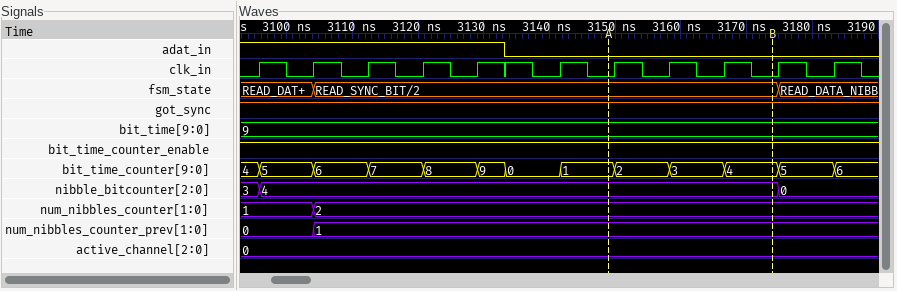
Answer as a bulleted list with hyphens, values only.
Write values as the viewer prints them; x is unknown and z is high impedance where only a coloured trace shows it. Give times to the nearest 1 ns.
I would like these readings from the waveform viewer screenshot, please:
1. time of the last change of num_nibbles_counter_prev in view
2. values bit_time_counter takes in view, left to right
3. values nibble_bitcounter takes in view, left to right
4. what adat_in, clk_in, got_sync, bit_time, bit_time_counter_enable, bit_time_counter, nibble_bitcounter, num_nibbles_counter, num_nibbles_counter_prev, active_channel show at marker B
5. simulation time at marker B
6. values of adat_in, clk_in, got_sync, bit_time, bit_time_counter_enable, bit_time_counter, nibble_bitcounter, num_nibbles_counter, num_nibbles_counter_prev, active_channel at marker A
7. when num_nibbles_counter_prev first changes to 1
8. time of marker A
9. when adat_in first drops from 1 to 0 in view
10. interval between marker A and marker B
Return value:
- 3104 ns
- 4, 5, 6, 7, 8, 9, 0, 1, 2, 3, 4, 5, 6
- 3, 4, 0
- adat_in=0, clk_in=0, got_sync=1, bit_time=9, bit_time_counter_enable=1, bit_time_counter=4, nibble_bitcounter=4, num_nibbles_counter=2, num_nibbles_counter_prev=1, active_channel=0
- 3174 ns
- adat_in=0, clk_in=0, got_sync=1, bit_time=9, bit_time_counter_enable=1, bit_time_counter=1, nibble_bitcounter=4, num_nibbles_counter=2, num_nibbles_counter_prev=1, active_channel=0
- 3104 ns
- 3149 ns
- 3133 ns
- 25 ns
